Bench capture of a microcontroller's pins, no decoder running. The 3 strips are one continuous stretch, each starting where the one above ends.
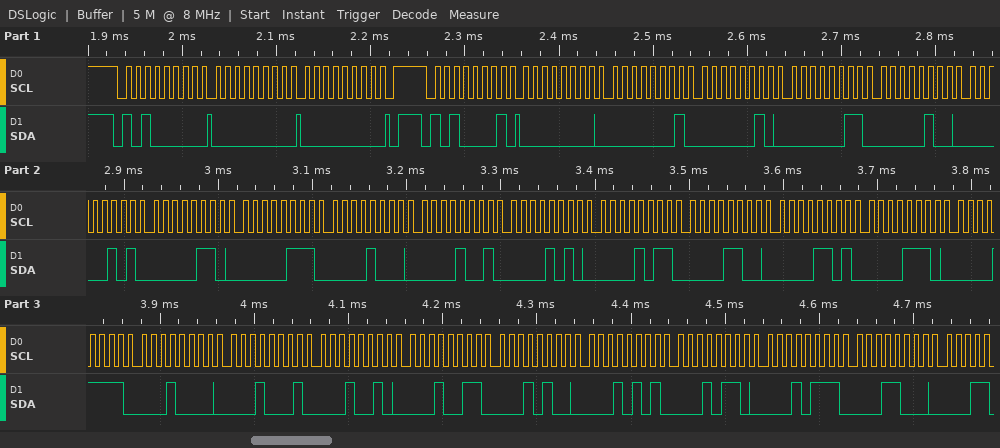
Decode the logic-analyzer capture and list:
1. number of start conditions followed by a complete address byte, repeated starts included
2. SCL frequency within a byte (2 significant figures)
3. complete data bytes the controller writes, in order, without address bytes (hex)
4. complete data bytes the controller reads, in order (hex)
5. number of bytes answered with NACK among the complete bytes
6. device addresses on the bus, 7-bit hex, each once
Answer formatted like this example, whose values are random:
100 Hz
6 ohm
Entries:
2
100 kHz
00 00
00 01 02 03 04 05 06 07 08 09 0A 0B 0C 0D 0E 0F 10 11 12 13 14 15 16 17 18
0
0x50
